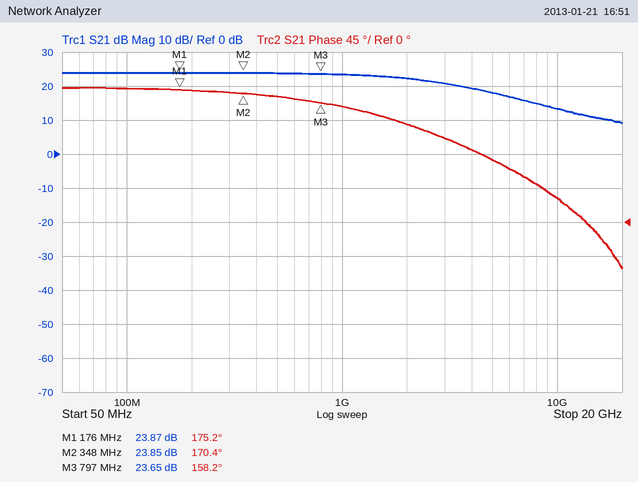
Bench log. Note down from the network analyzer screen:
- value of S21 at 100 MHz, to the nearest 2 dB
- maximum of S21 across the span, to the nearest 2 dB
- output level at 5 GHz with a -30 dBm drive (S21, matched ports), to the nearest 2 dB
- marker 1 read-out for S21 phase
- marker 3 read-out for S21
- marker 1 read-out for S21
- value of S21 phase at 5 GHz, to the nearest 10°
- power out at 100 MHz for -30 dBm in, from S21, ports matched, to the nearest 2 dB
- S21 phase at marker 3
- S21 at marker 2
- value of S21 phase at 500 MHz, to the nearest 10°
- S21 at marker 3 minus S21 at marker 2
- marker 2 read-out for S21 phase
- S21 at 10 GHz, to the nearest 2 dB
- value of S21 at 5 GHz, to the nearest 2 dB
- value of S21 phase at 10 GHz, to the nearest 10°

24 dB
24 dB
-12 dBm
175.2°
23.65 dB
23.87 dB
80°
-6 dBm
158.2°
23.85 dB
170°
-0.20 dB
170.4°
14 dB
18 dB
30°
